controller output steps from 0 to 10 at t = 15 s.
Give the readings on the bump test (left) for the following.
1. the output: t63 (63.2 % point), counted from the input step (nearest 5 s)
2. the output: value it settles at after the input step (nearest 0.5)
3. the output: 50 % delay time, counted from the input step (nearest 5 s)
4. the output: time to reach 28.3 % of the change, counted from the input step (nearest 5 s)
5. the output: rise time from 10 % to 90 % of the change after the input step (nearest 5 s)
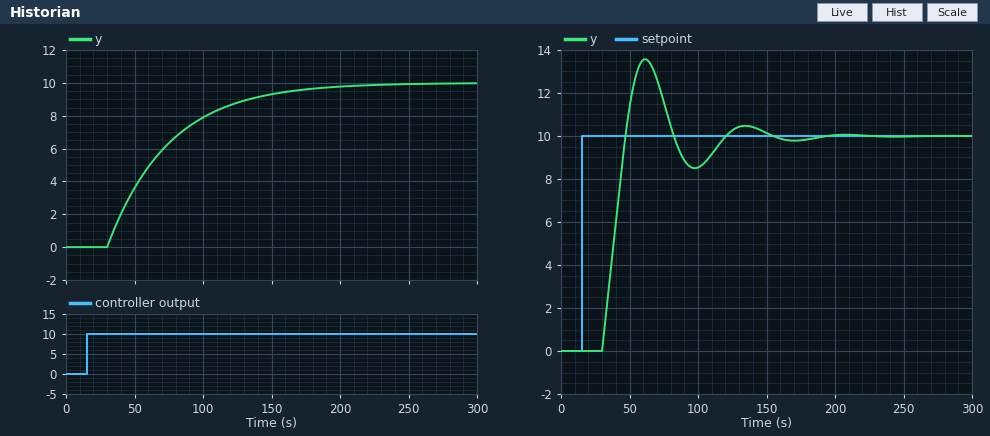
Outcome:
60 s
10.0
45 s
30 s
100 s
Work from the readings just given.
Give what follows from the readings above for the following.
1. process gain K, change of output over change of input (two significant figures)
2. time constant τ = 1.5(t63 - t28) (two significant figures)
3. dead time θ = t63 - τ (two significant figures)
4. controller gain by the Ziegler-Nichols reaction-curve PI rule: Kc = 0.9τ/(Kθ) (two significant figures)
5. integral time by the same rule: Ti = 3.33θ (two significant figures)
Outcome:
1.0
45 s
15 s
2.7
50 s
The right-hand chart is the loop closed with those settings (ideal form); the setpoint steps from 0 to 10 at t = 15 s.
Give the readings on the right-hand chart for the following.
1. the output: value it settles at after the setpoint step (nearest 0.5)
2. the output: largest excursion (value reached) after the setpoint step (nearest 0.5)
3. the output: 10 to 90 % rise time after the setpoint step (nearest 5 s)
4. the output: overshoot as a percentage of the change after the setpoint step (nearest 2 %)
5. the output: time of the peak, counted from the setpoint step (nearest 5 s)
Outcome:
10.0
13.5
15 s
36 %
45 s
